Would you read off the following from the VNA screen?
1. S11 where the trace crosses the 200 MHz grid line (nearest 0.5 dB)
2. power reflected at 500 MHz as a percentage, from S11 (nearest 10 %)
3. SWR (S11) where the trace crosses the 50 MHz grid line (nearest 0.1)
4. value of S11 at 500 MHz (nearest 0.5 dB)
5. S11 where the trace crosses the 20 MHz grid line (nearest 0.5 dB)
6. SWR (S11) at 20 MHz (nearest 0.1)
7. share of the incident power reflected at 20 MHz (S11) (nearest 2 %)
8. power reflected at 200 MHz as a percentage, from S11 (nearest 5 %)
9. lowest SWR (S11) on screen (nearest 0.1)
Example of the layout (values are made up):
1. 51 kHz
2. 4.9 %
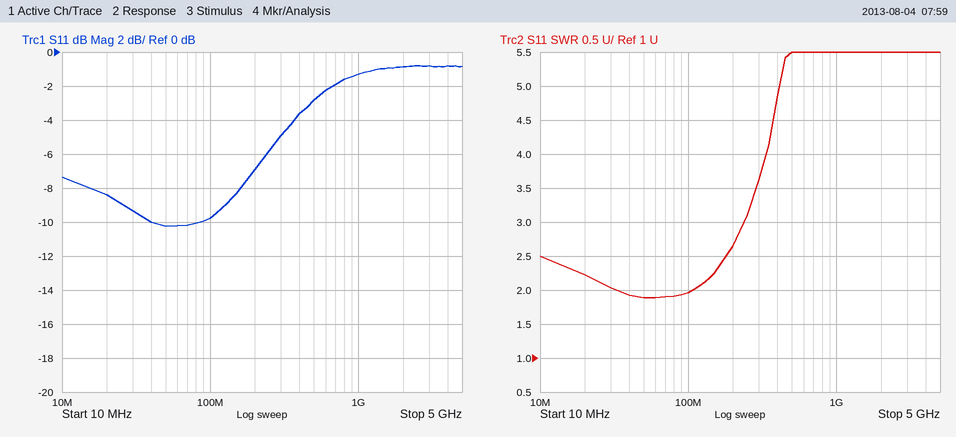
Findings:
1. -7.0 dB
2. 50 %
3. 1.9
4. -3.0 dB
5. -8.5 dB
6. 2.2
7. 14 %
8. 20 %
9. 1.9
